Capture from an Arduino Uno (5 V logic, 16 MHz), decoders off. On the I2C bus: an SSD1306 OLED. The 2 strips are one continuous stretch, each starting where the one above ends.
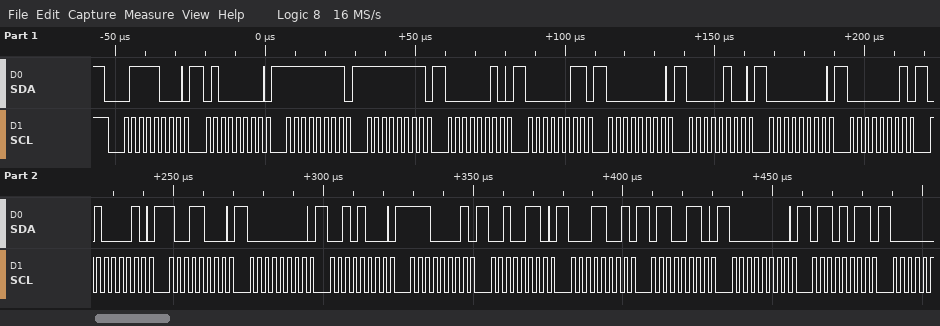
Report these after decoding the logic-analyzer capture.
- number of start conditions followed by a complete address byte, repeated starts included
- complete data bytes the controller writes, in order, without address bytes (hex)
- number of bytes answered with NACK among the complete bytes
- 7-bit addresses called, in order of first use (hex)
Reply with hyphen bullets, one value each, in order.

- 1
- 40 FF FF 02 03 00 04 00 01 42 98 00 28 E1 26 19 66 00 6B
- 0
- 0x3C
